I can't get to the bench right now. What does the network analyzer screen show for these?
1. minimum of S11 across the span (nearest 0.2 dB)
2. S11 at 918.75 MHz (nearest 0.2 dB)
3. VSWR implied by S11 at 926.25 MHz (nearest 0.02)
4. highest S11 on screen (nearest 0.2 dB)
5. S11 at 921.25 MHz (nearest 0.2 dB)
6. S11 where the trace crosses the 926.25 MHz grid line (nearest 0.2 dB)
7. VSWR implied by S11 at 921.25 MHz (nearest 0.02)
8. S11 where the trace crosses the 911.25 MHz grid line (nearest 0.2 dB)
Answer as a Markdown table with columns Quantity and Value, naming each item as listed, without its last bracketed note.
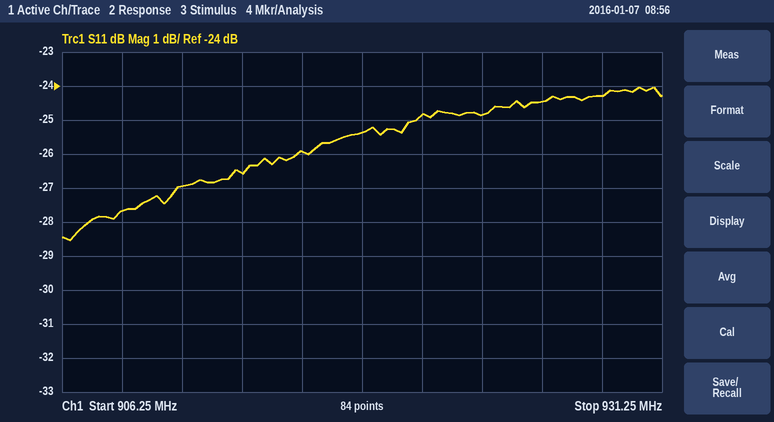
| Quantity | Value |
|---|---|
| minimum of S11 across the span | -28.6 dB |
| S11 at 918.75 MHz | -25.4 dB |
| VSWR implied by S11 at 926.25 MHz | 1.12 |
| highest S11 on screen | -24.0 dB |
| S11 at 921.25 MHz | -24.8 dB |
| S11 where the trace crosses the 926.25 MHz grid line | -24.4 dB |
| VSWR implied by S11 at 921.25 MHz | 1.12 |
| S11 where the trace crosses the 911.25 MHz grid line | -27.0 dB |
